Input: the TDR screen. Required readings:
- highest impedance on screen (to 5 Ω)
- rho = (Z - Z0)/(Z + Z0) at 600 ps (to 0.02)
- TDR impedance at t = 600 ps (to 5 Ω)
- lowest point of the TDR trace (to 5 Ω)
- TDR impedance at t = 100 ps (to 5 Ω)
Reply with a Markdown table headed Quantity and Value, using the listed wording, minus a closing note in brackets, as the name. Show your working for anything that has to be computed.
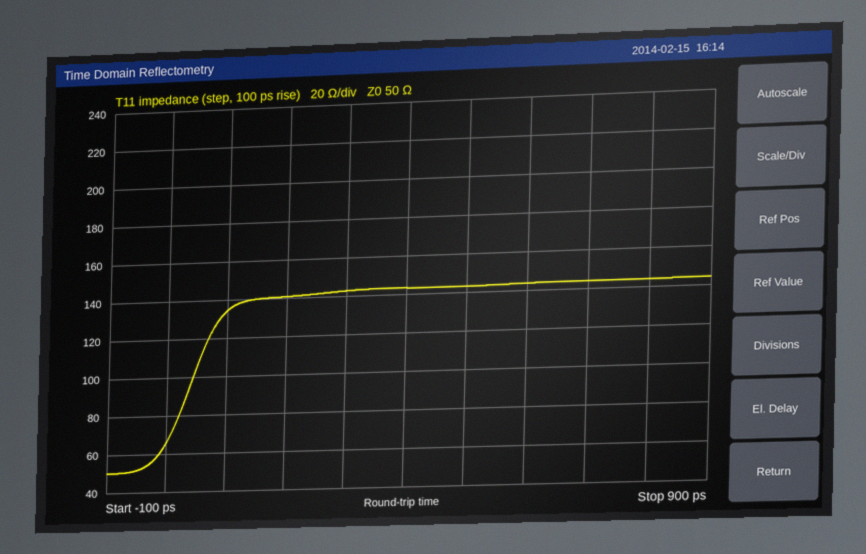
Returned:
| Quantity | Value |
|---|---|
| highest impedance on screen | 145 Ω |
| rho = (Z - Z0)/(Z + Z0) at 600 ps | (145 − 50)/(145 + 50) ≈ +0.487, so +0.48 to the nearest 0.02 |
| TDR impedance at t = 600 ps | 145 Ω |
| lowest point of the TDR trace | 50 Ω |
| TDR impedance at t = 100 ps | 135 Ω |
